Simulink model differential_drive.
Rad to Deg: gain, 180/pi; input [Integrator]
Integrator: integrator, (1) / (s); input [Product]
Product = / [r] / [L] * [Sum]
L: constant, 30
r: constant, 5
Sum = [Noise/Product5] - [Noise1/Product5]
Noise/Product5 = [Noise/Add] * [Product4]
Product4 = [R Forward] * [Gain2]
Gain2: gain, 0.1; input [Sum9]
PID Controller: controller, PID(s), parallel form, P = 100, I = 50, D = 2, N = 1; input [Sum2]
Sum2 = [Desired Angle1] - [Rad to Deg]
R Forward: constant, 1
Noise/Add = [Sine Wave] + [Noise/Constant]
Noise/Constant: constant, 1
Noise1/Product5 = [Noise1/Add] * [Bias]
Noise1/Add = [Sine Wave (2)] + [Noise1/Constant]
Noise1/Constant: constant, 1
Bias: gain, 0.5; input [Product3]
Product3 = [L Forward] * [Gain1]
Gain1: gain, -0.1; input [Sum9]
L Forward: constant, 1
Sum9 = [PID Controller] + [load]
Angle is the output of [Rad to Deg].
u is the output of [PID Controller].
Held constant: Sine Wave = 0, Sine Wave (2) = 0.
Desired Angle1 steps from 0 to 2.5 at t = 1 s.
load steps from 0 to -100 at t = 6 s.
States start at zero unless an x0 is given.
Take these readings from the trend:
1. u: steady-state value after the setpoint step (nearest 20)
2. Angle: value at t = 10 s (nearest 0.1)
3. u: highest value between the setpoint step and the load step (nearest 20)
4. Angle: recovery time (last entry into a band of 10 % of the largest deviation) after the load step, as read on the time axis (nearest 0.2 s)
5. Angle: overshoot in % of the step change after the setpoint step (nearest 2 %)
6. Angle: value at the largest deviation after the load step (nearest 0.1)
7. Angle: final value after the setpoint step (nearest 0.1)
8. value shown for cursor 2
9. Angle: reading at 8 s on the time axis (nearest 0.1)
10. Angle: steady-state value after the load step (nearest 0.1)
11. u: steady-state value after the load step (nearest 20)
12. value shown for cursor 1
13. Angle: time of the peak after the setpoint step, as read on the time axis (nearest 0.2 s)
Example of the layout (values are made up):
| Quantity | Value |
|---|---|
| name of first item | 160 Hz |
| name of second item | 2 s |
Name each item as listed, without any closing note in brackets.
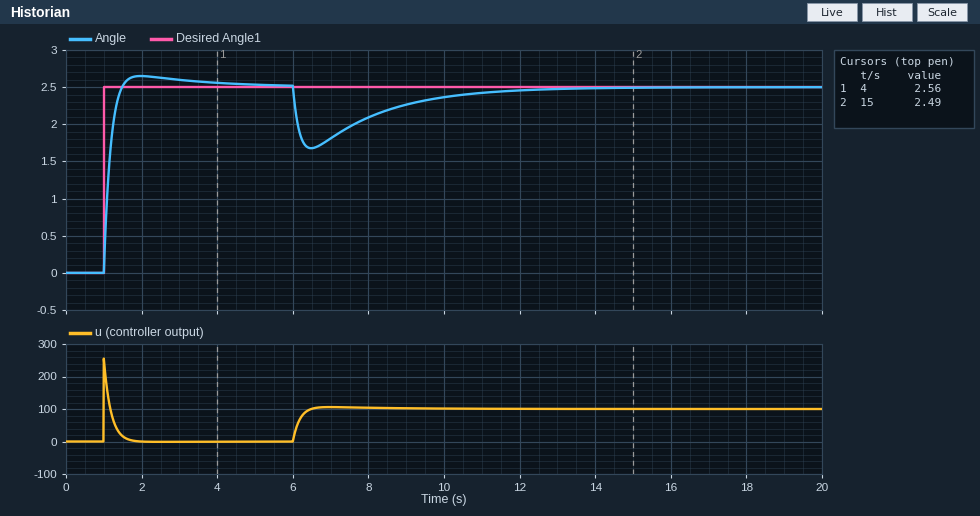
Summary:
| Quantity | Value |
|---|---|
| u: steady-state value after the setpoint step | 0 |
| Angle: value at t = 10 s | 2.4 |
| u: highest value between the setpoint step and the load step | 260 |
| Angle: recovery time (last entry into a band of 10 % of the largest deviation) after the load step, as read on the time axis | 10.8 s |
| Angle: overshoot in % of the step change after the setpoint step | 6 % |
| Angle: value at the largest deviation after the load step | 1.7 |
| Angle: final value after the setpoint step | 2.5 |
| value shown for cursor 2 | 2.49 |
| Angle: reading at 8 s on the time axis | 2.1 |
| Angle: steady-state value after the load step | 2.5 |
| u: steady-state value after the load step | 100 |
| value shown for cursor 1 | 2.56 |
| Angle: time of the peak after the setpoint step, as read on the time axis | 2.0 s |
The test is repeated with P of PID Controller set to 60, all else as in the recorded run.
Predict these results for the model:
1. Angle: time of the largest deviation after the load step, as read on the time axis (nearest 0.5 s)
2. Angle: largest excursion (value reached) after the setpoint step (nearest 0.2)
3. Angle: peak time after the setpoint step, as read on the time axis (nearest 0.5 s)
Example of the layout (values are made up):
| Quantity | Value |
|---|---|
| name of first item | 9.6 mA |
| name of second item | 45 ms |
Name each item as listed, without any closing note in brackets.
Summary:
| Quantity | Value |
|---|---|
| Angle: time of the largest deviation after the load step, as read on the time axis | 6.5 s |
| Angle: largest excursion (value reached) after the setpoint step | 2.8 |
| Angle: peak time after the setpoint step, as read on the time axis | 2.0 s |
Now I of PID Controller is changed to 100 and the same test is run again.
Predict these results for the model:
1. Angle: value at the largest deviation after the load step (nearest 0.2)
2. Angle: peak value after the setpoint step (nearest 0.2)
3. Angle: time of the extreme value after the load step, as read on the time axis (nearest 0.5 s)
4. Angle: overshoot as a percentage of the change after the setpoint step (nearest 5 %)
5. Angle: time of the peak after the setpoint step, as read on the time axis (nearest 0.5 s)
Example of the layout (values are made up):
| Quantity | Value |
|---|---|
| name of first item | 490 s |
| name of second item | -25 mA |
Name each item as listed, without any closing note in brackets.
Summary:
| Quantity | Value |
|---|---|
| Angle: value at the largest deviation after the load step | 1.8 |
| Angle: peak value after the setpoint step | 2.8 |
| Angle: time of the extreme value after the load step, as read on the time axis | 6.5 s |
| Angle: overshoot as a percentage of the change after the setpoint step | 10 % |
| Angle: time of the peak after the setpoint step, as read on the time axis | 2.0 s |
